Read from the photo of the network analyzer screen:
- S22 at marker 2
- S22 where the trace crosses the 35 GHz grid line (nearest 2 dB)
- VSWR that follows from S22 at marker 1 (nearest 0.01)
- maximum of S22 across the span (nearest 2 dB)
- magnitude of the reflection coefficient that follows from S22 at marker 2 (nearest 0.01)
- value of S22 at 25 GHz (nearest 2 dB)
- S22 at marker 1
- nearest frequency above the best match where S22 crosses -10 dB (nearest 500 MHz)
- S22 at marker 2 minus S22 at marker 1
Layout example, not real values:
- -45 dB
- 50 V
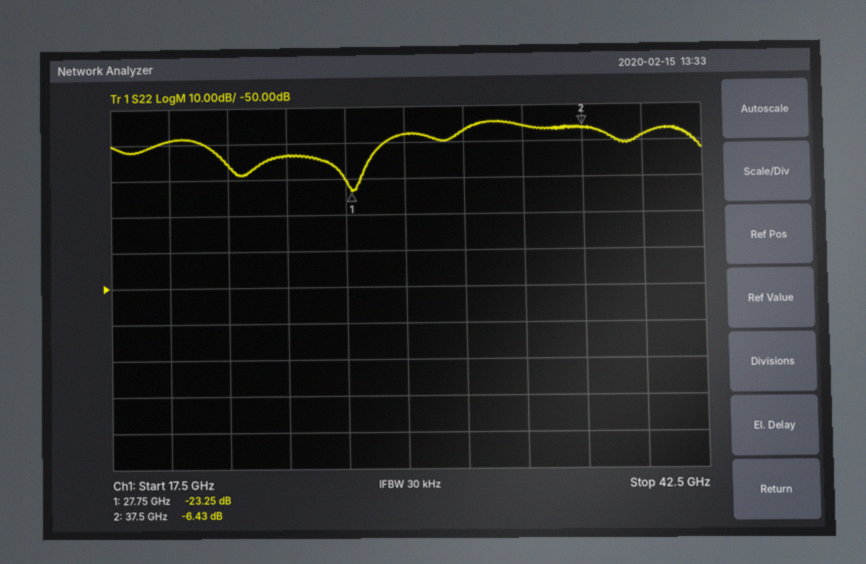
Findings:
- -6.43 dB
- -6 dB
- 1.15
- -4 dB
- 0.48
- -14 dB
- -23.25 dB
- 29.0 GHz
- 16.82 dB
